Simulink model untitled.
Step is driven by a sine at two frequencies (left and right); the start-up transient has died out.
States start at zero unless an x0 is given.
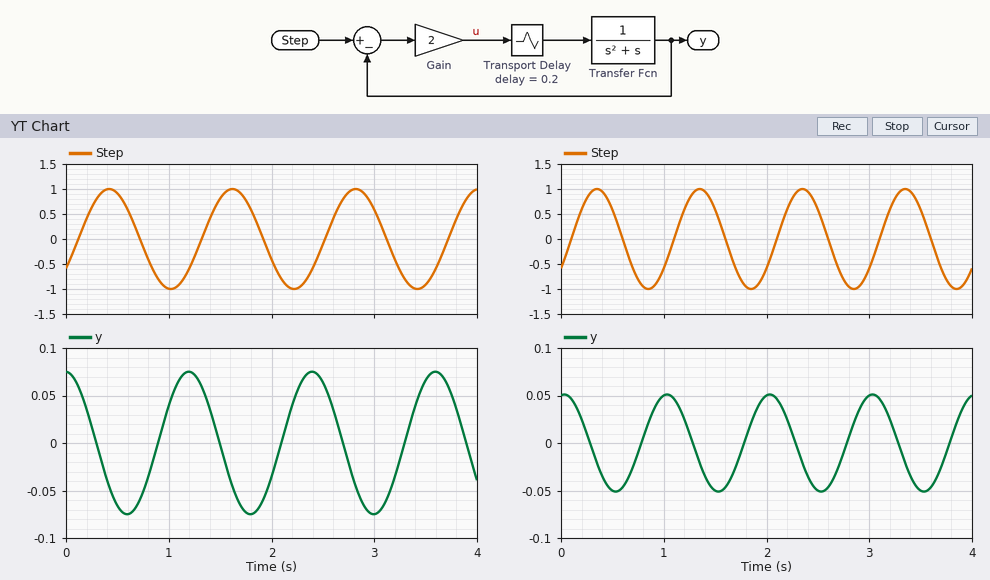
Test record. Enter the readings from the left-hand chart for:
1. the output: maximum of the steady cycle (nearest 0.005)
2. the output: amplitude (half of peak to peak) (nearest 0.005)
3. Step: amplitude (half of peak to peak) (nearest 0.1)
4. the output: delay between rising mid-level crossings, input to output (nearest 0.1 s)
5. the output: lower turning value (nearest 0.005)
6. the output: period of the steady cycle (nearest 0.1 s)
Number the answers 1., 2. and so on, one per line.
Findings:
1. 0.075
2. 0.075
3. 1.0
4. 0.8 s
5. -0.075
6. 1.2 s
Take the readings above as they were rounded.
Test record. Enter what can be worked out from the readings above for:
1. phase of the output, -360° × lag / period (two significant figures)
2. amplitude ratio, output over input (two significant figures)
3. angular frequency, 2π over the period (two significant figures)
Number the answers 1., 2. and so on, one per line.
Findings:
1. -240°
2. 0.075
3. 5.2 rad/s
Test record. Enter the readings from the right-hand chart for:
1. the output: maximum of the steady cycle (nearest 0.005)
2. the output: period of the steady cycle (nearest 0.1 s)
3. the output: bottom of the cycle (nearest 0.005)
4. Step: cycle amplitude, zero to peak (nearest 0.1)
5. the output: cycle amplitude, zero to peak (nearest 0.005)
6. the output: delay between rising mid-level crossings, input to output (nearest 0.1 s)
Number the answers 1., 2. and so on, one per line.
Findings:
1. 0.050
2. 1.0 s
3. -0.050
4. 1.0
5. 0.050
6. 0.7 s
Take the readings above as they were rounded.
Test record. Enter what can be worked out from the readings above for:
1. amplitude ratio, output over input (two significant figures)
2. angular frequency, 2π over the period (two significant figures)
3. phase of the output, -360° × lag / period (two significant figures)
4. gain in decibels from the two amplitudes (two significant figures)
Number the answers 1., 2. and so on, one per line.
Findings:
1. 0.050
2. 6.3 rad/s
3. -250°
4. -26 dB
